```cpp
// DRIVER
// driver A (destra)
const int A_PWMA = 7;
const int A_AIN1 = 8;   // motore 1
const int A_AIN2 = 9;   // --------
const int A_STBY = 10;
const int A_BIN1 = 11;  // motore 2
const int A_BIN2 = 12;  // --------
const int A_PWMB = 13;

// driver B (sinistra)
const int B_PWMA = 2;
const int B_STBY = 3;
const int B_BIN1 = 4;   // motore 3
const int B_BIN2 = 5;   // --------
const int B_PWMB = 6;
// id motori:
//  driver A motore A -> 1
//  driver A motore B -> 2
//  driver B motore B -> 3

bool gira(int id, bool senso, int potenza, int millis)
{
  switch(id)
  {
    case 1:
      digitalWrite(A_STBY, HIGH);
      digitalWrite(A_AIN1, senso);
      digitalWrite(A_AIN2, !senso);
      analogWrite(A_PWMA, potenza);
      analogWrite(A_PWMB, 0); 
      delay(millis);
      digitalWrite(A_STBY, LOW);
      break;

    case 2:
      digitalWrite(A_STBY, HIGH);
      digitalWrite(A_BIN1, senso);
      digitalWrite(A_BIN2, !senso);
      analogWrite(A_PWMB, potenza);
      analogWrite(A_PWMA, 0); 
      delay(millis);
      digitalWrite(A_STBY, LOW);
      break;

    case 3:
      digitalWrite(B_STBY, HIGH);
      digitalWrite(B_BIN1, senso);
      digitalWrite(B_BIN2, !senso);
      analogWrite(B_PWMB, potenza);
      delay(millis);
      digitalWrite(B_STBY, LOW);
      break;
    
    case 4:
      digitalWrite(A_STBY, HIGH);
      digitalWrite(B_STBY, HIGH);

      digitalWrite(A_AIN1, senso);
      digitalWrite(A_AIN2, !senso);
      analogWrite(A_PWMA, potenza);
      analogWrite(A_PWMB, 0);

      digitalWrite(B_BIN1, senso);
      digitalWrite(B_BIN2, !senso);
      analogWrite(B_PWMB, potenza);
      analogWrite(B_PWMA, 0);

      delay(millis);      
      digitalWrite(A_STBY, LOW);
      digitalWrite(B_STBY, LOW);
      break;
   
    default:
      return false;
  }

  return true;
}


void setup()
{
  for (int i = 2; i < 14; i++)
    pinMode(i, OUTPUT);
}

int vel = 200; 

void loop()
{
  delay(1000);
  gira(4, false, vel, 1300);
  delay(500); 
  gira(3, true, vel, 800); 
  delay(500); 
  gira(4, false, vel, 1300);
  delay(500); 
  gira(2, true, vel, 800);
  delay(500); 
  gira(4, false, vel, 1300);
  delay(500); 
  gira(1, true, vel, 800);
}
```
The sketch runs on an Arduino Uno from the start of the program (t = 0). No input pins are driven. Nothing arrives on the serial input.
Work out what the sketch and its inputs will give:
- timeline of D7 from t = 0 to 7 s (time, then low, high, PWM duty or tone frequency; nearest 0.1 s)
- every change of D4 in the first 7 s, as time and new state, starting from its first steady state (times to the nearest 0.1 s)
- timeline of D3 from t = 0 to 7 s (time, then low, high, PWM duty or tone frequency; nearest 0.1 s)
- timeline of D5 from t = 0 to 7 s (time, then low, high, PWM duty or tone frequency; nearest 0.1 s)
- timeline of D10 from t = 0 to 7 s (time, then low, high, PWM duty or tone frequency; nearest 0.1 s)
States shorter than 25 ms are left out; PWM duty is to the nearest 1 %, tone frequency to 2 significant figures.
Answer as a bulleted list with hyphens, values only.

- 0 s low; 1 s high; 5.9 s low
- 0 s low; 2.8 s high; 4.1 s low
- 0 s low; 1 s high; 2.3 s low; 2.8 s high; 3.6 s low; 4.1 s high; 5.4 s low
- 0 s low; 1 s high; 2.8 s low; 4.1 s high
- 0 s low; 1 s high; 2.3 s low; 4.1 s high; 5.4 s low; 5.9 s high; 6.7 s low
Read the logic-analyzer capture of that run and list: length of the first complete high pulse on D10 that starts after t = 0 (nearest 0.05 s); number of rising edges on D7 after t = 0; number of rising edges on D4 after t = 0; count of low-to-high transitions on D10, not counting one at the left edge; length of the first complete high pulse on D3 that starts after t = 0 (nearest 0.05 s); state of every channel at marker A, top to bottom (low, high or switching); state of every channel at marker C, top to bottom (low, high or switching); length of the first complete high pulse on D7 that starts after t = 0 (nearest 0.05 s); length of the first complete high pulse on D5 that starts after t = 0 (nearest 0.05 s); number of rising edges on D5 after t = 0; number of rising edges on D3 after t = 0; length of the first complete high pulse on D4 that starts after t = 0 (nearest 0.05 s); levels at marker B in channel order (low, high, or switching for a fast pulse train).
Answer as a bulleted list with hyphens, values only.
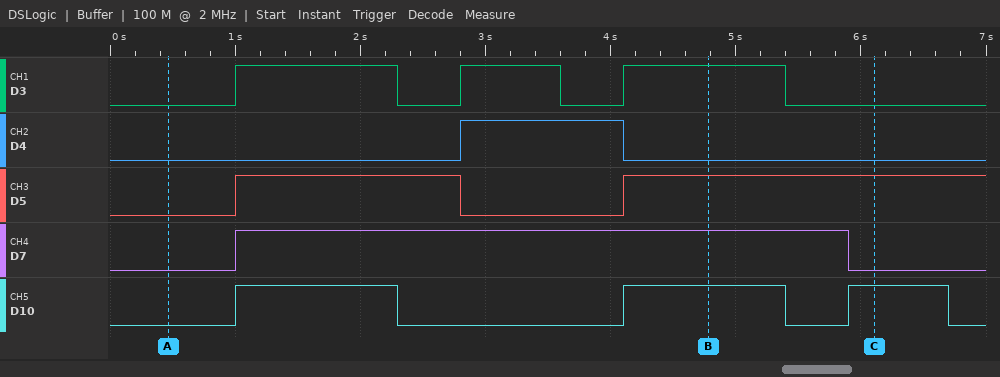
- 1.30 s
- 1
- 1
- 3
- 1.30 s
- D3 low, D4 low, D5 low, D7 low, D10 low
- D3 low, D4 low, D5 high, D7 low, D10 high
- 4.90 s
- 1.80 s
- 2
- 3
- 1.30 s
- D3 high, D4 low, D5 high, D7 high, D10 high
